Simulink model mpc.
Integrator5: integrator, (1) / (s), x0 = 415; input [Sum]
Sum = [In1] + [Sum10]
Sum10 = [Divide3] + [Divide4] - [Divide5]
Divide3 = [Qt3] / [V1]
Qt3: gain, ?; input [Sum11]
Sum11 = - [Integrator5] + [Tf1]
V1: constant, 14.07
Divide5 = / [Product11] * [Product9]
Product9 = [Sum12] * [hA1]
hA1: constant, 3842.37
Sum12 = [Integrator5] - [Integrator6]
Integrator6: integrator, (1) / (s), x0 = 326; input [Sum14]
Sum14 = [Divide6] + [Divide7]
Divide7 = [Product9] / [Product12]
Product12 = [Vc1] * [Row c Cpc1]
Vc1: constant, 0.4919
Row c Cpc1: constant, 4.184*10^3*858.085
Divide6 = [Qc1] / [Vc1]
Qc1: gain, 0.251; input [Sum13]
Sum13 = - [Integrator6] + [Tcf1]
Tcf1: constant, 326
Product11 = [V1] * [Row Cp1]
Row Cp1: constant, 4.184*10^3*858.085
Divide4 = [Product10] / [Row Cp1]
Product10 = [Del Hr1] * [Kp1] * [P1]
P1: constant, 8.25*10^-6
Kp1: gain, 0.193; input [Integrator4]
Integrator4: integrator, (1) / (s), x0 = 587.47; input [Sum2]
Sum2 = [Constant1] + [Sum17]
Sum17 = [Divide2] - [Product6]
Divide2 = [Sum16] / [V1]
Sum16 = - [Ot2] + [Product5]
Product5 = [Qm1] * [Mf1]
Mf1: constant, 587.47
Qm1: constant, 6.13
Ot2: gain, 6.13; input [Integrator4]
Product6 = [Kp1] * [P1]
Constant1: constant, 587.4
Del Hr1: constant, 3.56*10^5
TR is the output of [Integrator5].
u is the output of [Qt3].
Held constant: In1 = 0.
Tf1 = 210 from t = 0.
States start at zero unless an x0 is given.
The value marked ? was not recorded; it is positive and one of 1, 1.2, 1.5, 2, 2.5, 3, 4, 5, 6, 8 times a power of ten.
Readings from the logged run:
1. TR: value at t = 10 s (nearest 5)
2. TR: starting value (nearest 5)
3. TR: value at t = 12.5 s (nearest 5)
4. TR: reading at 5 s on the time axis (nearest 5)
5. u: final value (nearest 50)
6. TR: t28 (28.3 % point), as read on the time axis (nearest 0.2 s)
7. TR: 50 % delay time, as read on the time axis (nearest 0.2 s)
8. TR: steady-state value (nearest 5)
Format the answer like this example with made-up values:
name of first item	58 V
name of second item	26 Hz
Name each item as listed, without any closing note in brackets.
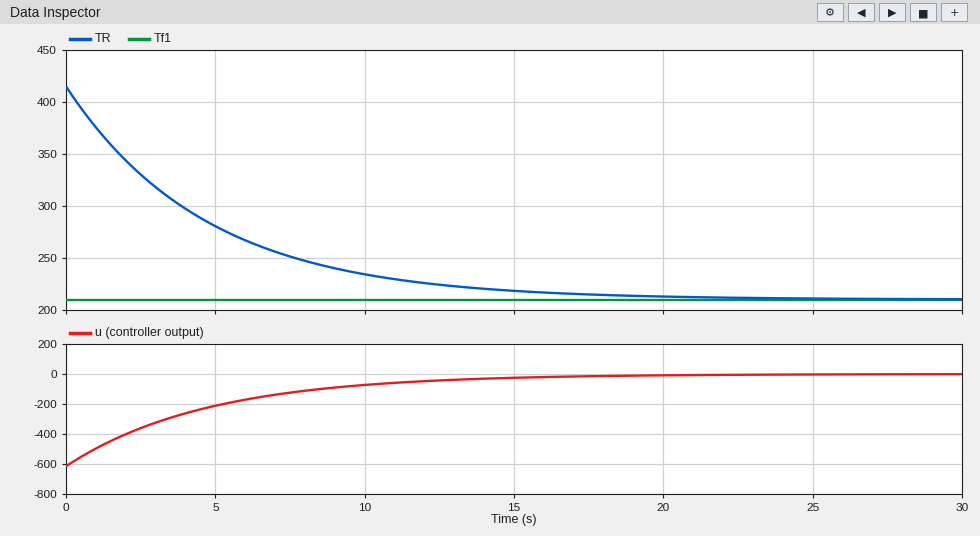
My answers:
TR: value at t = 10 s	235
TR: starting value	415
TR: value at t = 12.5 s	225
TR: reading at 5 s on the time axis	280
u: final value	0
TR: t28 (28.3 % point), as read on the time axis	1.6 s
TR: 50 % delay time, as read on the time axis	3.2 s
TR: steady-state value	210
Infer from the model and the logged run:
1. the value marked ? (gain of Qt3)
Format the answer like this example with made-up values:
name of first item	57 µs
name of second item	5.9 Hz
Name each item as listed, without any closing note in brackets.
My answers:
the value marked ?	3
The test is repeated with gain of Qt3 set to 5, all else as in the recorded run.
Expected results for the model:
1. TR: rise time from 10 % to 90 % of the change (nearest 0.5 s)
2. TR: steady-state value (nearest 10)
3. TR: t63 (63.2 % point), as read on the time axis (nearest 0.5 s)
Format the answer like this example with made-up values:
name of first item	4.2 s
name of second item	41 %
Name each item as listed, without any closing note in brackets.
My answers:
TR: rise time from 10 % to 90 % of the change	6.0 s
TR: steady-state value	210
TR: t63 (63.2 % point), as read on the time axis	3.0 s
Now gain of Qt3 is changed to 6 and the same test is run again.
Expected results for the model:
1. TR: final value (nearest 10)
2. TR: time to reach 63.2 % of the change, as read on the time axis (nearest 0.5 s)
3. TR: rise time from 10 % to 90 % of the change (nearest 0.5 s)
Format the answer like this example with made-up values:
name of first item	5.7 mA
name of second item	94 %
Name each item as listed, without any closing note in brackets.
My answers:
TR: final value	210
TR: time to reach 63.2 % of the change, as read on the time axis	2.5 s
TR: rise time from 10 % to 90 % of the change	5.0 s
